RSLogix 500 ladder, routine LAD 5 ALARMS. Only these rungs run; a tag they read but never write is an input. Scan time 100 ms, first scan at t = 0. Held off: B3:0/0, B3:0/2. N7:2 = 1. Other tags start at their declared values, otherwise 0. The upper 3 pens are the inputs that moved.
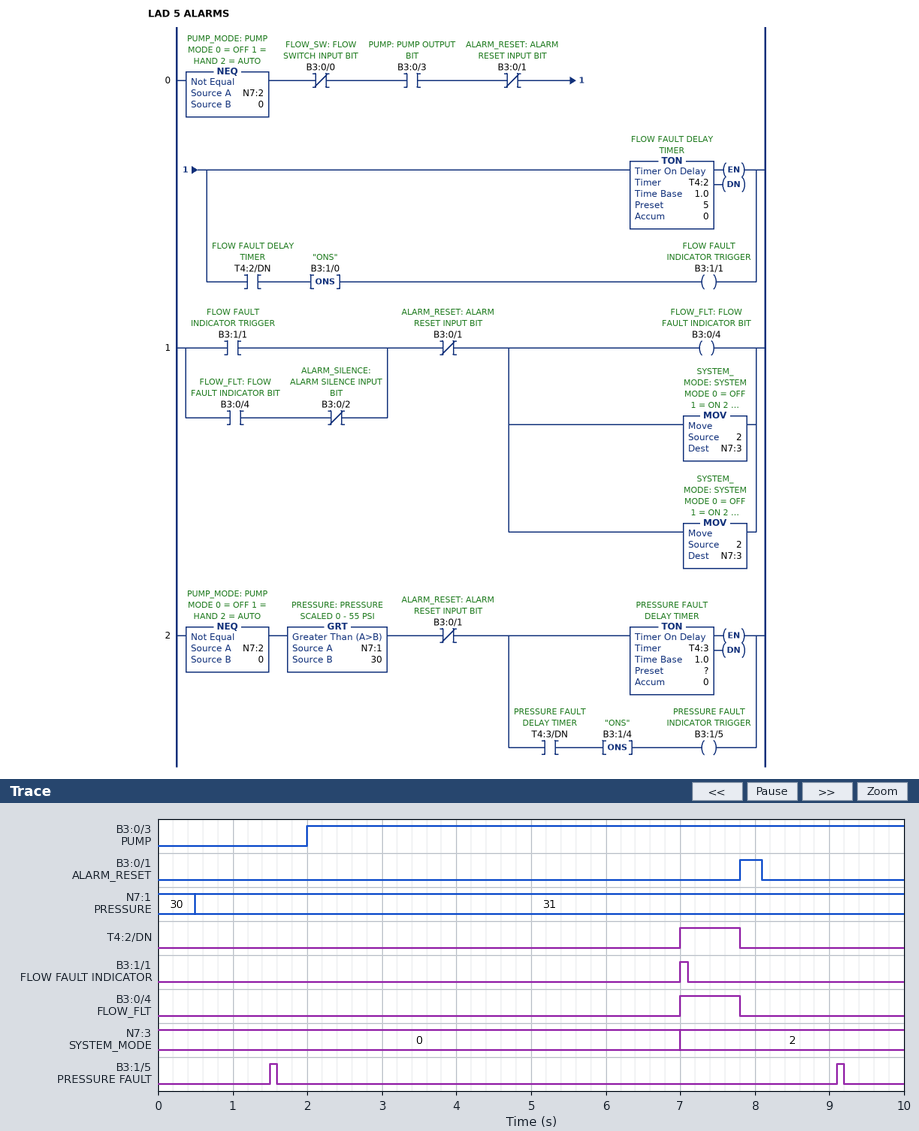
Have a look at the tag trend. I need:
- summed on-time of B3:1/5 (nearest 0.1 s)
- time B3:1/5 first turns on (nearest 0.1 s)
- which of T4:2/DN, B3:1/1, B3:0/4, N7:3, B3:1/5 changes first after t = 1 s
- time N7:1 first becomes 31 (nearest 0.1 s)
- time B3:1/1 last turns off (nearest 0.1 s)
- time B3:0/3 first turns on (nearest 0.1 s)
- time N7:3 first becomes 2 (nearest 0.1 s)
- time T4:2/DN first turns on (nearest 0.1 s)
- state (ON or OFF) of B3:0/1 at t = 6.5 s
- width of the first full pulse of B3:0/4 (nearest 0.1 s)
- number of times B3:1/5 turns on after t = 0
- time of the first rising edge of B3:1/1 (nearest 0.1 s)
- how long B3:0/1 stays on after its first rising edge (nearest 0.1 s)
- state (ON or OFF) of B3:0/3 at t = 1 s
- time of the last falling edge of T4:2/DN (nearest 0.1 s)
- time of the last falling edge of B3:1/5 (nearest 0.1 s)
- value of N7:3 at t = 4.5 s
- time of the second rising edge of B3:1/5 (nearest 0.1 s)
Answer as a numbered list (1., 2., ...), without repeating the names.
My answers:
1. 0.2 s
2. 1.5 s
3. B3:1/5
4. 0.5 s
5. 7.1 s
6. 2.0 s
7. 7.0 s
8. 7.0 s
9. OFF
10. 0.8 s
11. 2
12. 7.0 s
13. 0.3 s
14. OFF
15. 7.8 s
16. 9.2 s
17. 0
18. 9.1 s
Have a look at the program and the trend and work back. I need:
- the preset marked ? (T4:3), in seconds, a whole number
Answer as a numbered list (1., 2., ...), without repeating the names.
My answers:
1. 1 s
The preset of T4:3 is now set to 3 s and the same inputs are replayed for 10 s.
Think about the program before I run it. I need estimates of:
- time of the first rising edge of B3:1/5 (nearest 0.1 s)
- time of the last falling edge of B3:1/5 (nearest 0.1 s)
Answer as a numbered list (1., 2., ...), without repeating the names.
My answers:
1. 3.5 s
2. 3.6 s
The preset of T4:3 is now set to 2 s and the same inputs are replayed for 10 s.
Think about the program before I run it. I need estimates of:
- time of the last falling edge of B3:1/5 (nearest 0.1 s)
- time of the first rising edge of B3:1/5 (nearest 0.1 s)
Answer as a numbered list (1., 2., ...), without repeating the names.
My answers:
1. 2.6 s
2. 2.5 s
